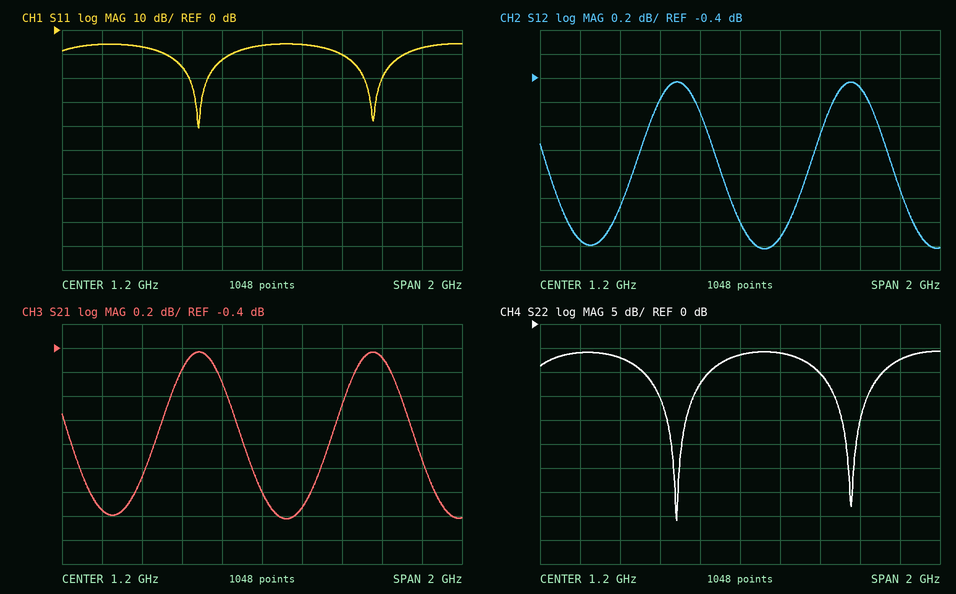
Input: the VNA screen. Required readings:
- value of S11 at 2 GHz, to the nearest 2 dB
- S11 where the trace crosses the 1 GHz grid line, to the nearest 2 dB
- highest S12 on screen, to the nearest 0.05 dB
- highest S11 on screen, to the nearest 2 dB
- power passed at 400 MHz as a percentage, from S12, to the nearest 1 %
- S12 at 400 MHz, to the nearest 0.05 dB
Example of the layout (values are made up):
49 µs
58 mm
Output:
-8 dB
-12 dB
-0.45 dB
-6 dB
67 %
-1.75 dB
